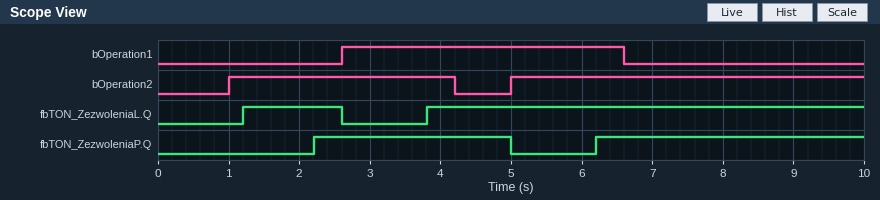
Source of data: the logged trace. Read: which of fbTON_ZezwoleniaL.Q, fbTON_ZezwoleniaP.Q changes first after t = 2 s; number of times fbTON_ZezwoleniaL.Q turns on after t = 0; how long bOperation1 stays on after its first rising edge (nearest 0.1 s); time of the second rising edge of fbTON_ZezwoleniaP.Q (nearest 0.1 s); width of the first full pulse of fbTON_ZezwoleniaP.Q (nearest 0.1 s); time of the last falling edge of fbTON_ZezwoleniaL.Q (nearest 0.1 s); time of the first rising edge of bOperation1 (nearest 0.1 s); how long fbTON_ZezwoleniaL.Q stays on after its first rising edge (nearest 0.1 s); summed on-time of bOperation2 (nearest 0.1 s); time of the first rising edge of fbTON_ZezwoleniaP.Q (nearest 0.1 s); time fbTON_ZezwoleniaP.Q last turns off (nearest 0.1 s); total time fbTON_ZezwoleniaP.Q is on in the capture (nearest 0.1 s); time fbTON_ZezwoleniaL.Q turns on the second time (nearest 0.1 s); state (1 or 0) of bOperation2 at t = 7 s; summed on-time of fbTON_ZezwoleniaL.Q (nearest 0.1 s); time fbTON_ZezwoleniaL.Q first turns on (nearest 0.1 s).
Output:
fbTON_ZezwoleniaP.Q
2
4.0 s
6.2 s
2.8 s
2.6 s
2.6 s
1.4 s
8.2 s
2.2 s
5.0 s
6.6 s
3.8 s
1
7.6 s
1.2 s
